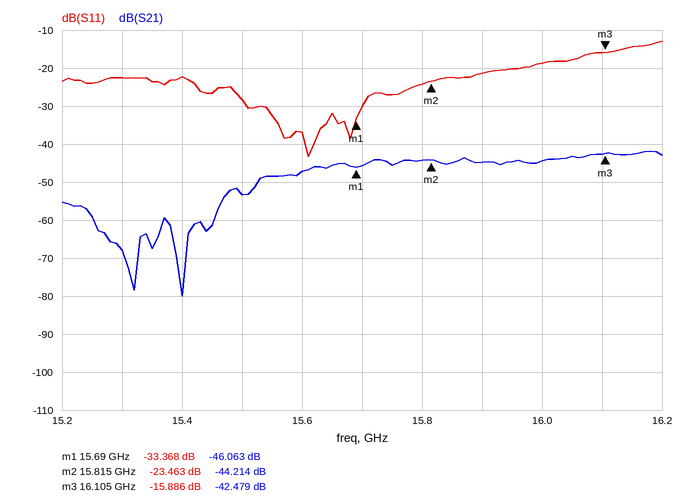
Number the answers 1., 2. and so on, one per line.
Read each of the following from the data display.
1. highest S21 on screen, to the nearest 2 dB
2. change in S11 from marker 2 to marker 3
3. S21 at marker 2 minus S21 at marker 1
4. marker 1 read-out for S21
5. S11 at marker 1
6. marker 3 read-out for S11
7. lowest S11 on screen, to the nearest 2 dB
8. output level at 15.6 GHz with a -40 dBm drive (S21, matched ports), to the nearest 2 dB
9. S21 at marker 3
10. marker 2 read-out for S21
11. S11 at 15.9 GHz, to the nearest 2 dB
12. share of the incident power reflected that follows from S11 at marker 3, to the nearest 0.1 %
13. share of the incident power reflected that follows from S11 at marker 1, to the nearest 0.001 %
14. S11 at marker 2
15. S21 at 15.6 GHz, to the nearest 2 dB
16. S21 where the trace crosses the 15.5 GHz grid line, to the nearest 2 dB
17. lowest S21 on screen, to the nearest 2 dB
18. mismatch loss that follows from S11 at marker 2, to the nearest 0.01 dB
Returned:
1. -42 dB
2. 7.577 dB
3. 1.849 dB
4. -46.063 dB
5. -33.368 dB
6. -15.886 dB
7. -44 dB
8. -88 dBm
9. -42.479 dB
10. -44.214 dB
11. -22 dB
12. 2.6 %
13. 0.046 %
14. -23.463 dB
15. -48 dB
16. -54 dB
17. -80 dB
18. 0.02 dB
